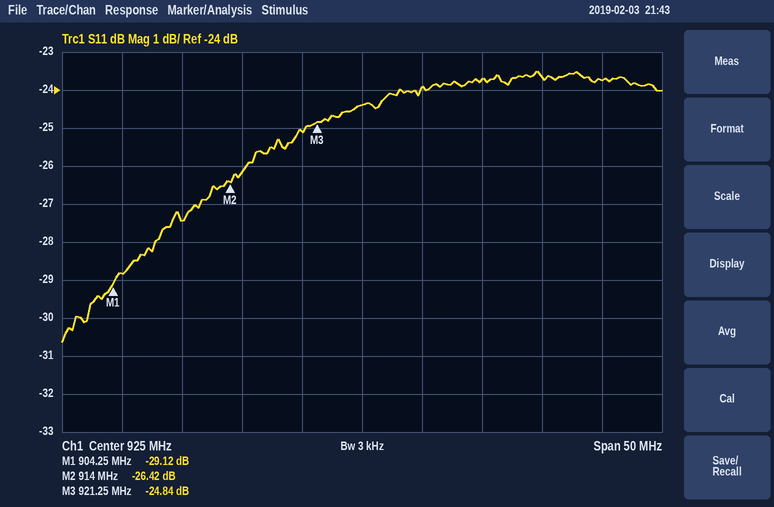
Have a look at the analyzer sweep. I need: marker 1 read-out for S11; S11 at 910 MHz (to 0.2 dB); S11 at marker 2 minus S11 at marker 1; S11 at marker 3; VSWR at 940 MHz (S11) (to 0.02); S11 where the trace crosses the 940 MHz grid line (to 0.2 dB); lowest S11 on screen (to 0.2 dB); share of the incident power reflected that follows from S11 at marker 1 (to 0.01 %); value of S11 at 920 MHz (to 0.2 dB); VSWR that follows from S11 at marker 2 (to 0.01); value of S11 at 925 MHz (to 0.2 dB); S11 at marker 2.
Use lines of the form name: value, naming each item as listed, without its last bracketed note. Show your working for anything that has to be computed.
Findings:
marker 1 read-out for S11: -29.12 dB
S11 at 910 MHz: -27.4 dB
S11 at marker 2 minus S11 at marker 1: -26.42 − (-29.12) = 2.70 dB
S11 at marker 3: -24.84 dB
VSWR at 940 MHz (S11): |Γ| = 10^(-23.6/20) = 0.0661; VSWR = (1 + 0.0661)/(1 − 0.0661) ≈ 1.14
S11 where the trace crosses the 940 MHz grid line: -23.6 dB
lowest S11 on screen: -30.6 dB
share of the incident power reflected that follows from S11 at marker 1: 10^(-29.12/10) ≈ 0.12 %
value of S11 at 920 MHz: -25.0 dB
VSWR that follows from S11 at marker 2: (1 + 0.0478)/(1 − 0.0478) ≈ 1.10
value of S11 at 925 MHz: -24.4 dB
S11 at marker 2: -26.42 dB
